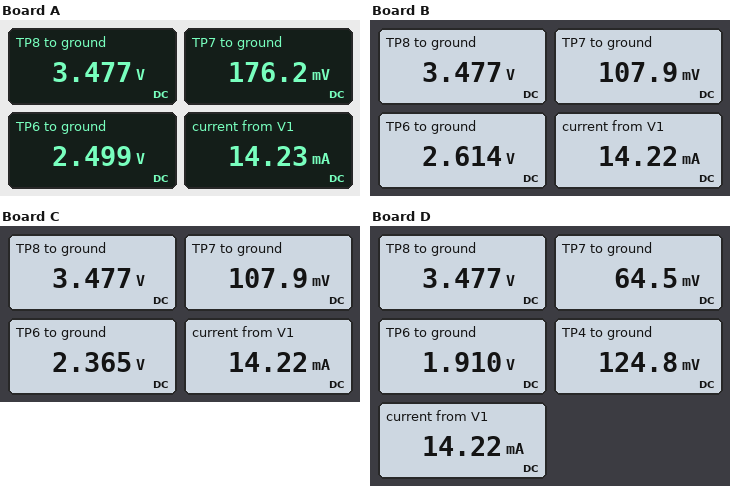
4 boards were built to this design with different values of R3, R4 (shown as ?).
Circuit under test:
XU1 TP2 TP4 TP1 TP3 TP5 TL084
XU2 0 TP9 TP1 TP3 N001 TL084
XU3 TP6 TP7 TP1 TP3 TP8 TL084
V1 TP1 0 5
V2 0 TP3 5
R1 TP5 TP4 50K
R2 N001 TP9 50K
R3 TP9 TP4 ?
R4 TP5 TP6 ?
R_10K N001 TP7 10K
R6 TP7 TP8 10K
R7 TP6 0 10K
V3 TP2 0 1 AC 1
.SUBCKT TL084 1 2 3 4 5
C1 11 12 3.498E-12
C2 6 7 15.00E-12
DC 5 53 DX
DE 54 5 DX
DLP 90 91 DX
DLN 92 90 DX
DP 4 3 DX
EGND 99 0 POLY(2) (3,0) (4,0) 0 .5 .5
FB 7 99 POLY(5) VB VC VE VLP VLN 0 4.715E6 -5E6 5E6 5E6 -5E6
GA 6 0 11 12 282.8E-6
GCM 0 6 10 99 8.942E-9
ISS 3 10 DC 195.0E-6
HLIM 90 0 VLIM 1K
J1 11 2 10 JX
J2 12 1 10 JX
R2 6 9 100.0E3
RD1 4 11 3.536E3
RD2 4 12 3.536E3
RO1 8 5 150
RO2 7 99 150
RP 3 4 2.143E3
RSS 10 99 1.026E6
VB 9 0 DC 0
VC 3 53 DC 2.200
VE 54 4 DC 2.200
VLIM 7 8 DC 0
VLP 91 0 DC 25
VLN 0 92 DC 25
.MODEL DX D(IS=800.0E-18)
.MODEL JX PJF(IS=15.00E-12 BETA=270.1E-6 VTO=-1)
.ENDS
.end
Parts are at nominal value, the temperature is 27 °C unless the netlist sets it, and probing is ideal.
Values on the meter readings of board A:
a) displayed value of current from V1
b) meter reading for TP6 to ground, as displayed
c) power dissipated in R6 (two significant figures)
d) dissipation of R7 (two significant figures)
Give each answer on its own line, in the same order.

14.23 mA
2.499 V
1.1 mW
620 µW
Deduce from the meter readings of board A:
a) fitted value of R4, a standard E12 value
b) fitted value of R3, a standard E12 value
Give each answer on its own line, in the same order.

3.9 kΩ
5.6 kΩ
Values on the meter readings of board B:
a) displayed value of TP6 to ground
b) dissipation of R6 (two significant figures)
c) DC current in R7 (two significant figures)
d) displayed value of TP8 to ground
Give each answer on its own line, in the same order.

2.614 V
1.1 mW
260 µA
3.477 V
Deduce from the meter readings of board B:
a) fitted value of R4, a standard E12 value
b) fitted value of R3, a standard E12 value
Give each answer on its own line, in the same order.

3.3 kΩ
3.3 kΩ
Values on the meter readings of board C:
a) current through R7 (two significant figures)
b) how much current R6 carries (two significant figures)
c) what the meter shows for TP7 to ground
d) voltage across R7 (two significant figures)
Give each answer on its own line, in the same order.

240 µA
340 µA
107.9 mV
2.4 V
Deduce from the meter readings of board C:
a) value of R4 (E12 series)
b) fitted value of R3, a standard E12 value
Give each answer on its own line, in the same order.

4.7 kΩ
3.3 kΩ
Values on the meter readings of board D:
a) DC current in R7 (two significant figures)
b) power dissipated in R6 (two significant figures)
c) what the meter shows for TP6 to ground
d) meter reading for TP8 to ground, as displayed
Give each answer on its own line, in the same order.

190 µA
1.2 mW
1.910 V
3.477 V
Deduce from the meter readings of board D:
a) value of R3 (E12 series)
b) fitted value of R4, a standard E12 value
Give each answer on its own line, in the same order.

1.8 kΩ
8.2 kΩ
